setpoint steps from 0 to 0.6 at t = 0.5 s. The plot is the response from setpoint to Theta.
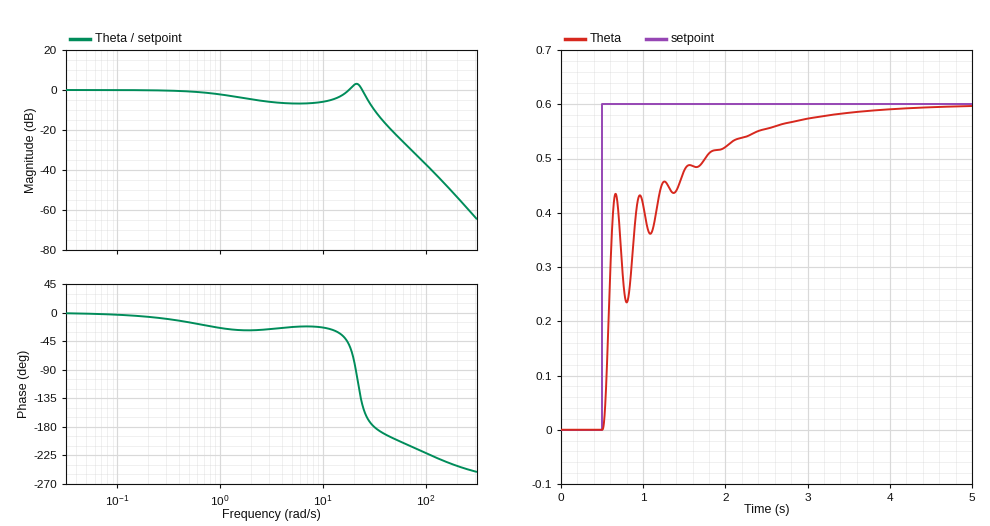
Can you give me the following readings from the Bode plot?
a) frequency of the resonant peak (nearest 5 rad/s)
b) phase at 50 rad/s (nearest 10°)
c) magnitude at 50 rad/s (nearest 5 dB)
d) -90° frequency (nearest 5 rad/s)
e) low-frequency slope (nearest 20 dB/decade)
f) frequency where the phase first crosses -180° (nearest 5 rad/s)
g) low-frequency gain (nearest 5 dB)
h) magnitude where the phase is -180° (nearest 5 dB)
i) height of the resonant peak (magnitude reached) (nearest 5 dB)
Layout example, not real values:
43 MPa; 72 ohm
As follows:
20 rad/s; -200°; -20 dB; 20 rad/s; 0 dB/decade; 30 rad/s; 0 dB; -10 dB; 5 dB
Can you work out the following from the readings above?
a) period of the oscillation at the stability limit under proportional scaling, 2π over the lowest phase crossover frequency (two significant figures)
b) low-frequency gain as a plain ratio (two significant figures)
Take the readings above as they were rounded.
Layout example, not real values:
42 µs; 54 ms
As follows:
0.21 s; 1.0
